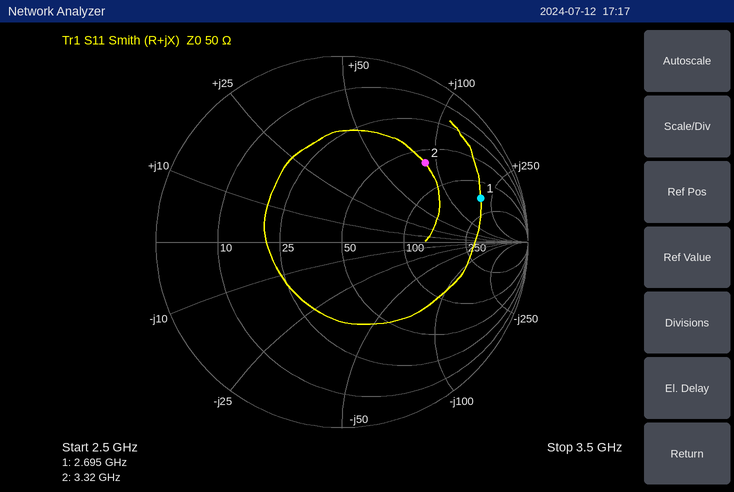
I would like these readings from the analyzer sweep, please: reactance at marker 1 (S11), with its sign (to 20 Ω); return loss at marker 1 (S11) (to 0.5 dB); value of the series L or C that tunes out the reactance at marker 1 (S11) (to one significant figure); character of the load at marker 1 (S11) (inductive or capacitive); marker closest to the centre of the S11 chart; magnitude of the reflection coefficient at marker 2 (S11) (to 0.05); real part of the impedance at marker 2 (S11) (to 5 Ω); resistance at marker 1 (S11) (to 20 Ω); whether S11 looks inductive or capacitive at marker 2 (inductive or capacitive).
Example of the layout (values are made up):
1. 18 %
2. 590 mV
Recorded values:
1. +200 Ω
2. 2.0 dB
3. 300 fF
4. inductive
5. marker 2
6. 0.60
7. 65 Ω
8. 160 Ω
9. inductive
